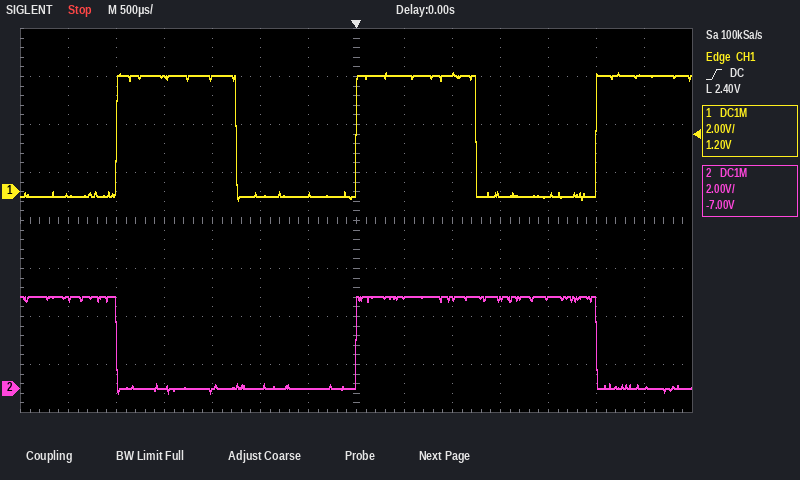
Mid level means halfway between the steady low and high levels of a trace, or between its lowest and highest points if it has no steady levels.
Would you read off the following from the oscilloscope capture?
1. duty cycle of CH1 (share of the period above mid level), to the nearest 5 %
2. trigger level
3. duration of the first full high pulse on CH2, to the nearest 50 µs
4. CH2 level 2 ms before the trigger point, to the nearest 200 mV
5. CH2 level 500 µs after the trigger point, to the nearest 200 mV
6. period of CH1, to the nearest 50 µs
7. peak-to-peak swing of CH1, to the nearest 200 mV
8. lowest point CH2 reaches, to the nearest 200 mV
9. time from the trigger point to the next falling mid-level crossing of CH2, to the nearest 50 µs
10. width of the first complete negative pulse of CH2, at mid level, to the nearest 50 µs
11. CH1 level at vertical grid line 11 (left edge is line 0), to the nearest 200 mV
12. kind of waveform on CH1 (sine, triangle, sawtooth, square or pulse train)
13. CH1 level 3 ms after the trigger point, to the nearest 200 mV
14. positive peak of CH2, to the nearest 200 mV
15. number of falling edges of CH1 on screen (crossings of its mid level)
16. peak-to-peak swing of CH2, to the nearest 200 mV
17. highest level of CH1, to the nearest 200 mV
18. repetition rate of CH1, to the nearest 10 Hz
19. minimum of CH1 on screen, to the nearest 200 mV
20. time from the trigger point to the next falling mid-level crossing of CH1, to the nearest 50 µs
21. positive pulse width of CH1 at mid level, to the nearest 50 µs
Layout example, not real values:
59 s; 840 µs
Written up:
50 %; 2.40 V; 2.50 ms; 0.0 V; 3.8 V; 2.50 ms; 5.4 V; -200 mV; 2.50 ms; 2.50 ms; -200 mV; square; 4.8 V; 3.8 V; 2; 4.0 V; 5.0 V; 400 Hz; -400 mV; 1.25 ms; 1.25 ms
